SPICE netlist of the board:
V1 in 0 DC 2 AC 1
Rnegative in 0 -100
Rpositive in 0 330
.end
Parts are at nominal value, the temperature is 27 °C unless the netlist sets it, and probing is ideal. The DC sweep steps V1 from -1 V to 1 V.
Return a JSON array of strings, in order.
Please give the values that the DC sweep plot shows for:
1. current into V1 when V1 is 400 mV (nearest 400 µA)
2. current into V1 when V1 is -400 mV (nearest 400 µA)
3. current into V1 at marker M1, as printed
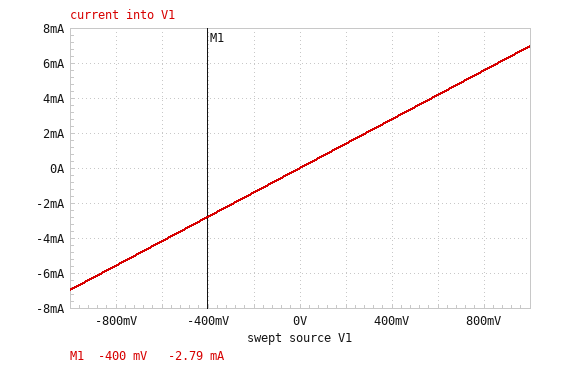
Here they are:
["2.8 mA", "-2.8 mA", "-2.79 mA"]
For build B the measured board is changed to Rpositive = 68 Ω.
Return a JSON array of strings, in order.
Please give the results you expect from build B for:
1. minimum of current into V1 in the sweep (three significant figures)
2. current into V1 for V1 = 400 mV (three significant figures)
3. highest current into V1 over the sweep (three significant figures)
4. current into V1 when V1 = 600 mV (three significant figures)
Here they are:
["-4.71 mA", "-1.88 mA", "4.71 mA", "-2.82 mA"]
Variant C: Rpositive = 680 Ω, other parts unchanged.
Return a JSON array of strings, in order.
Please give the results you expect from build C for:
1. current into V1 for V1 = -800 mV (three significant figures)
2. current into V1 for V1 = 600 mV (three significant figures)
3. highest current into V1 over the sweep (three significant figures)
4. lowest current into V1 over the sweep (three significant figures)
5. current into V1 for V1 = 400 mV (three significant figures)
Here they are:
["-6.82 mA", "5.12 mA", "8.53 mA", "-8.53 mA", "3.41 mA"]
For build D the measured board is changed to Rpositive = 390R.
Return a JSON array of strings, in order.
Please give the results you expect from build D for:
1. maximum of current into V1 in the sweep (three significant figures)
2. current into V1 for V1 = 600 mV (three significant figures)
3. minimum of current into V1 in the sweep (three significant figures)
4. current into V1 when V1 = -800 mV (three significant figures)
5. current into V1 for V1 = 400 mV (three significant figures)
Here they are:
["7.44 mA", "4.46 mA", "-7.44 mA", "-5.95 mA", "2.97 mA"]
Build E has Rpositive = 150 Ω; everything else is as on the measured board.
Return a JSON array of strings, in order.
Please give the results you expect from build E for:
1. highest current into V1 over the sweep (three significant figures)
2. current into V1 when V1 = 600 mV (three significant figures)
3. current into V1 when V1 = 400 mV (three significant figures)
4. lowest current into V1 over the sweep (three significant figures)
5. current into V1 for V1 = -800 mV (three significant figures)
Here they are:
["3.33 mA", "2.00 mA", "1.33 mA", "-3.33 mA", "-2.67 mA"]
